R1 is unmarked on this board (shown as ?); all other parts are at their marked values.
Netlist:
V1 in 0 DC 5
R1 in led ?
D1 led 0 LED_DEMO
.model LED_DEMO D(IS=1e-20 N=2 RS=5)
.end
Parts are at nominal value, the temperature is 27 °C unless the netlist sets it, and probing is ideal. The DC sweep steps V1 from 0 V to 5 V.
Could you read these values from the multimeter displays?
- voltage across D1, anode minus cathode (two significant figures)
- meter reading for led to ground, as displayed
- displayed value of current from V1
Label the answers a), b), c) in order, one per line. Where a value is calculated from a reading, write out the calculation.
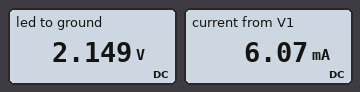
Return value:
a) 2.149 V = 2.1 V
b) 2.149 V
c) 6.07 mA
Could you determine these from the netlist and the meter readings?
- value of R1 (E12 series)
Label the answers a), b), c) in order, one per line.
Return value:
a) 470 Ω
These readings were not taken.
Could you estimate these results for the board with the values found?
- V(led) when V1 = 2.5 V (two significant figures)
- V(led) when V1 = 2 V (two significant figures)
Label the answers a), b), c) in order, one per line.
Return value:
a) 2.0 V
b) 1.9 V
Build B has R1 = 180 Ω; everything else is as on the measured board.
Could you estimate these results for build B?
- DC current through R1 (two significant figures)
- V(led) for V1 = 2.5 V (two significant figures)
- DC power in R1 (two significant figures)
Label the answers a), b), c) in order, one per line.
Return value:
a) 15 mA
b) 2.1 V
c) 42 mW
